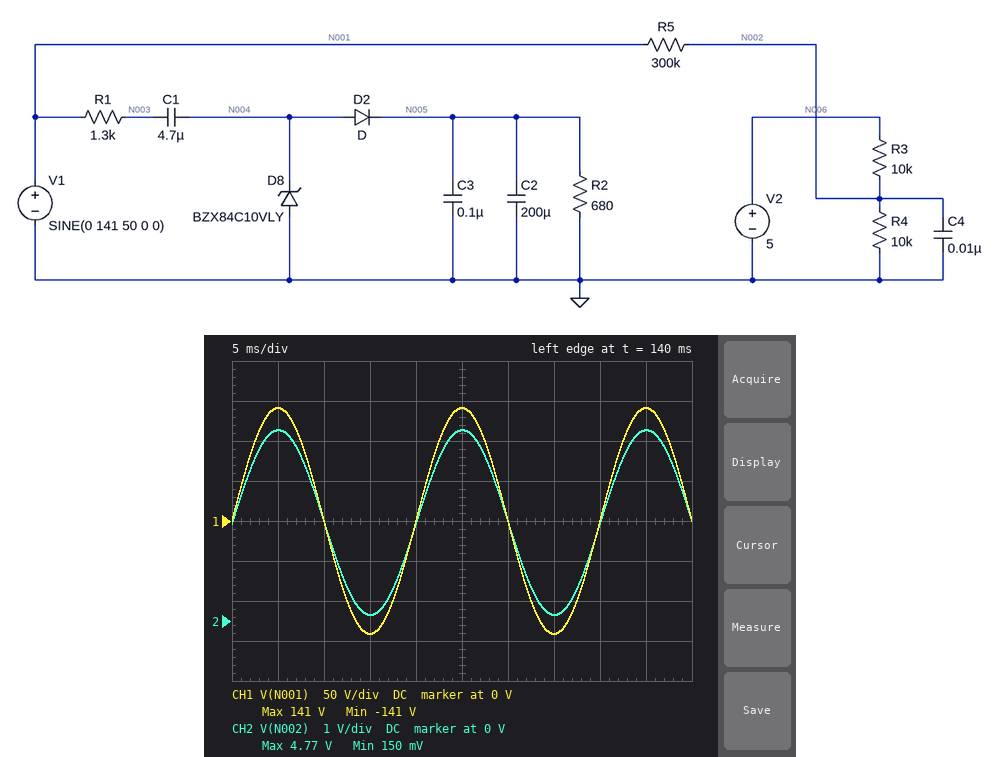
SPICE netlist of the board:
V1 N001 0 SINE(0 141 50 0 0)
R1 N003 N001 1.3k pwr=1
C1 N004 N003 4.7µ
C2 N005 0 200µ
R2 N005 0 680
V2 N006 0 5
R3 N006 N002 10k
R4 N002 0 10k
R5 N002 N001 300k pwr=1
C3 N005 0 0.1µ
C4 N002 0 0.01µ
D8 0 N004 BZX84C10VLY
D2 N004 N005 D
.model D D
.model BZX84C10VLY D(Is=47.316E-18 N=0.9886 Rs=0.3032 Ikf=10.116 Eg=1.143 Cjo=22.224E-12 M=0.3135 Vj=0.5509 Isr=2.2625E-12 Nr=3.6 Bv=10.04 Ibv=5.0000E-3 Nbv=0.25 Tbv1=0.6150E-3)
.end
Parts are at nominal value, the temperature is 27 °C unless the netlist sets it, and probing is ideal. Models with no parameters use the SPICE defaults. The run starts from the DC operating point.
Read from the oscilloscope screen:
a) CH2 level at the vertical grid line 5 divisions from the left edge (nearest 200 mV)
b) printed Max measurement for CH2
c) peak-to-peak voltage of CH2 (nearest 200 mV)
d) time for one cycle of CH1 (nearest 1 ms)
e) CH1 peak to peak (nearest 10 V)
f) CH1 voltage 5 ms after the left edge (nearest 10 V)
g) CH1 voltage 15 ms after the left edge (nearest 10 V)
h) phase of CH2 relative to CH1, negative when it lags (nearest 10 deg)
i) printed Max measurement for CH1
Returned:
4.8 V
4.77 V
4.6 V
20 ms
280 V
140 V
-140 V
0 deg
141 V
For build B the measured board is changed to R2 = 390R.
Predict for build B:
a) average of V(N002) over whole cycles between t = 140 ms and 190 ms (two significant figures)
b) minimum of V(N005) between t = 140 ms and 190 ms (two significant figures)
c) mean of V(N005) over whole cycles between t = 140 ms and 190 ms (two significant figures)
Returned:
2.5 V
8.1 V
8.8 V
